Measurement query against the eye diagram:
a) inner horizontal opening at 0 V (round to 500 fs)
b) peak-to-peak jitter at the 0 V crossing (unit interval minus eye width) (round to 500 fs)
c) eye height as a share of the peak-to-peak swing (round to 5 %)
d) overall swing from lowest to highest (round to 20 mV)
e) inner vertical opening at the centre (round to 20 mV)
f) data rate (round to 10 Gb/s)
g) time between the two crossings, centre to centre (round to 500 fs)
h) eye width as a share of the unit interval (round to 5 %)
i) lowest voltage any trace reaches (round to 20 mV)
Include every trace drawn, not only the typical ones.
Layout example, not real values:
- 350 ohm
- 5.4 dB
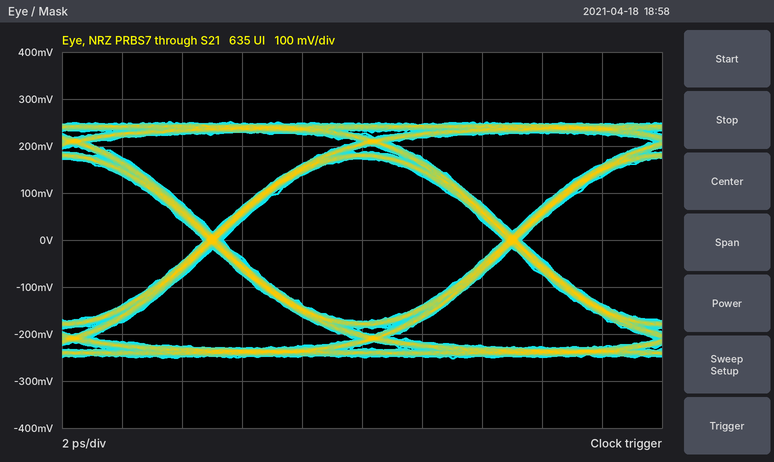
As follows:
- 9.5 ps
- 500 fs
- 70 %
- 500 mV
- 340 mV
- 100 Gb/s
- 10.0 ps
- 95 %
- -260 mV
